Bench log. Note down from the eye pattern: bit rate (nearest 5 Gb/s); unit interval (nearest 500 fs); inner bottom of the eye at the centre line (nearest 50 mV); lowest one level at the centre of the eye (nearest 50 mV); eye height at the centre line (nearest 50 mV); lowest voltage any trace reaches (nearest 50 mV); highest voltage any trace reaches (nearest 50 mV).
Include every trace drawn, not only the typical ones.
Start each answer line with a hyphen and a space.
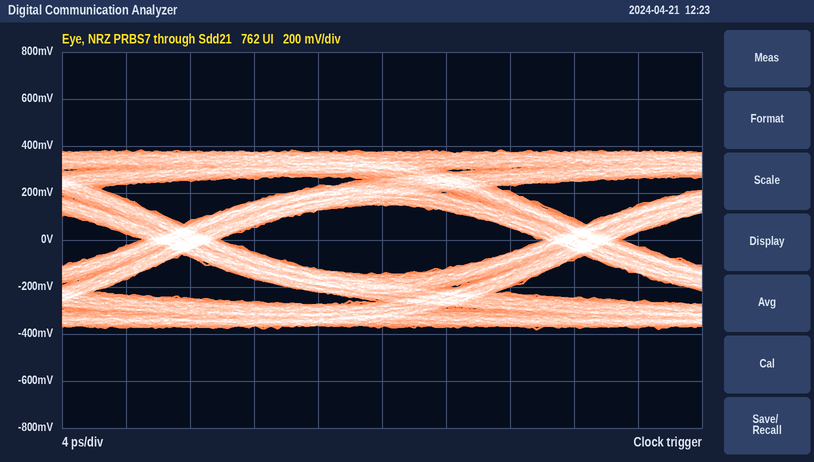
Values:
- 40 Gb/s
- 25.0 ps
- -150 mV
- 150 mV
- 300 mV
- -400 mV
- 400 mV
